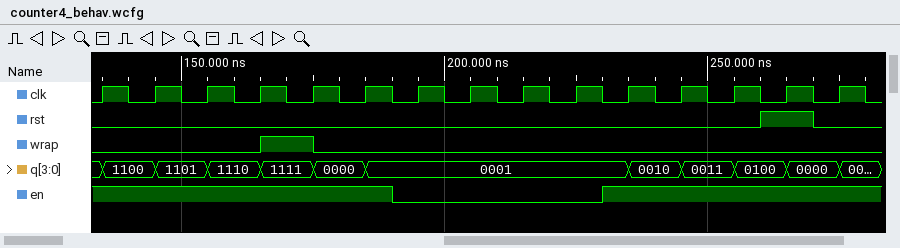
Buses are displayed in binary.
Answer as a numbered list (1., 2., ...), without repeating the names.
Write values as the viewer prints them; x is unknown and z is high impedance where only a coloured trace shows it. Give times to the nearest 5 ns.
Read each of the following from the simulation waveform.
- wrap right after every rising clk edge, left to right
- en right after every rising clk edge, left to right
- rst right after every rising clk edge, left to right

1. 0 0 0 1 0 0 0 0 0 0 0 0 0 0 0
2. 1 1 1 1 1 1 0 0 0 0 1 1 1 1 1
3. 0 0 0 0 0 0 0 0 0 0 0 0 0 1 0
